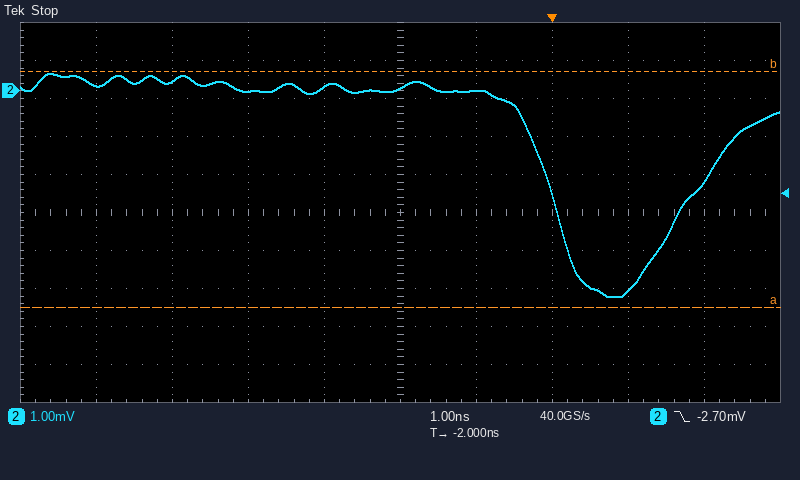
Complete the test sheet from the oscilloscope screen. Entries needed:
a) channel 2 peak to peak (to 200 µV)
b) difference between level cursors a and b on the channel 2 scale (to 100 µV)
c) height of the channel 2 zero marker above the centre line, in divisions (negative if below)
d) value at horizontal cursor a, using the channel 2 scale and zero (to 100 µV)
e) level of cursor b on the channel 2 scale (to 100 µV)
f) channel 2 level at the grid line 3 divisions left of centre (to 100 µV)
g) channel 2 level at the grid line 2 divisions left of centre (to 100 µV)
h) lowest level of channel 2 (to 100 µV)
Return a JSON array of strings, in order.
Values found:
["5.8 mV", "6.2 mV", "+3.2 div", "-5.7 mV", "500 µV", "300 µV", "0.0 mV", "-5.4 mV"]
